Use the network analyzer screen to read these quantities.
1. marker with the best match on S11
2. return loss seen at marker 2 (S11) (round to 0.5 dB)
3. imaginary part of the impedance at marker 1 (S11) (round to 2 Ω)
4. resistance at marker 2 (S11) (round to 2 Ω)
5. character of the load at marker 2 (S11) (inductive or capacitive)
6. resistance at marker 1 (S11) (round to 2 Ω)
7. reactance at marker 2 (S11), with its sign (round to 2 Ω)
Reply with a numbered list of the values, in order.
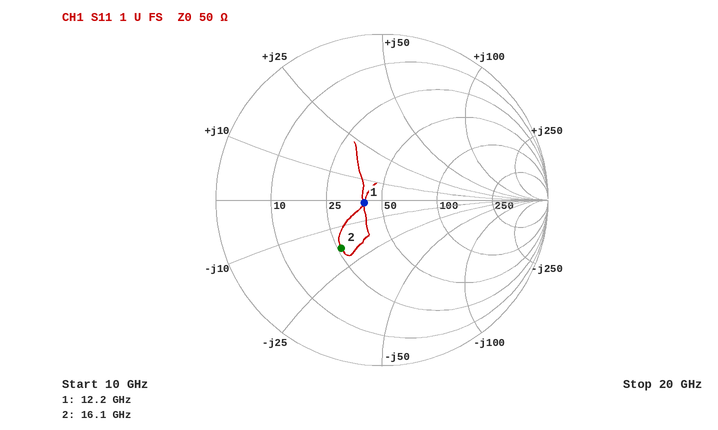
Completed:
1. marker 1
2. 8.5 dB
3. -2 Ω
4. 26 Ω
5. capacitive
6. 40 Ω
7. -18 Ω
